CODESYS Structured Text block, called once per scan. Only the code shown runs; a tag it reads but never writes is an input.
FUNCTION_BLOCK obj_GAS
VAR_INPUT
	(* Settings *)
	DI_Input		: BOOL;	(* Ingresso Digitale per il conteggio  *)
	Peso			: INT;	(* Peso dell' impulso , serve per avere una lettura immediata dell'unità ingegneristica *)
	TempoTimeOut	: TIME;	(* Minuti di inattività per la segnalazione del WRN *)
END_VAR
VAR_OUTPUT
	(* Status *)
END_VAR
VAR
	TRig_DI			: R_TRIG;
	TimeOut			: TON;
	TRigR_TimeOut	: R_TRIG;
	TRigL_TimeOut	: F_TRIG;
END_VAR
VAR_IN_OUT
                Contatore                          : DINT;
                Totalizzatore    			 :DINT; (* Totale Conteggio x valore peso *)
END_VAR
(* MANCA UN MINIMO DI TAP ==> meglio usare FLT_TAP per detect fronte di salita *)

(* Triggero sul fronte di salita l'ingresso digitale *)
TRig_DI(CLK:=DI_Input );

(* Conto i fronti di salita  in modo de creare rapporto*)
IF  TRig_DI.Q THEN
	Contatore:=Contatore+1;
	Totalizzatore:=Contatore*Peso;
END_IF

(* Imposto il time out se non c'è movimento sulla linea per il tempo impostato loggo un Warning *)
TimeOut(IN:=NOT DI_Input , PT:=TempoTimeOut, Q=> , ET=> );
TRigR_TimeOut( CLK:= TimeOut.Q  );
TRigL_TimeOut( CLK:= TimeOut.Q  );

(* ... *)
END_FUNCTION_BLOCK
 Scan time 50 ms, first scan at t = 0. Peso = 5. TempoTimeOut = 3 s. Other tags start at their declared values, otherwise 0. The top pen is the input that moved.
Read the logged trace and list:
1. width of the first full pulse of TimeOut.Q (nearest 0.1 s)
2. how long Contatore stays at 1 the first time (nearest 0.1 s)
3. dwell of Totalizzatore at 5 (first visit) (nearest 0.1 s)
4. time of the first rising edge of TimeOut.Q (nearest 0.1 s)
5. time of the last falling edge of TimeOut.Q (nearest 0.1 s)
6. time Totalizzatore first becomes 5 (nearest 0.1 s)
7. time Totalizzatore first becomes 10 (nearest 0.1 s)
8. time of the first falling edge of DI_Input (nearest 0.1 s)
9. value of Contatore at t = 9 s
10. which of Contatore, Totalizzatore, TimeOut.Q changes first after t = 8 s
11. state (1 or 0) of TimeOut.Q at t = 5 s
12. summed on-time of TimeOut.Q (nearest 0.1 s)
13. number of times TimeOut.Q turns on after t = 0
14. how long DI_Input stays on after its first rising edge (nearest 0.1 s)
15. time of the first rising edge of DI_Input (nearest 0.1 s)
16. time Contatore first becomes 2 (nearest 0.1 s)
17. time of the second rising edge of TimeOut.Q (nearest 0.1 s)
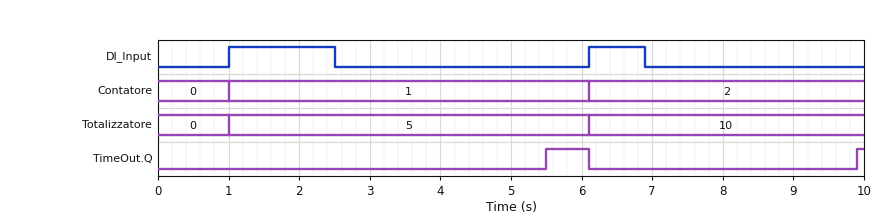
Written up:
0.6 s
5.1 s
5.1 s
5.5 s
6.1 s
1.0 s
6.1 s
2.5 s
2
TimeOut.Q
0
0.7 s
2
1.5 s
1.0 s
6.1 s
9.9 s
